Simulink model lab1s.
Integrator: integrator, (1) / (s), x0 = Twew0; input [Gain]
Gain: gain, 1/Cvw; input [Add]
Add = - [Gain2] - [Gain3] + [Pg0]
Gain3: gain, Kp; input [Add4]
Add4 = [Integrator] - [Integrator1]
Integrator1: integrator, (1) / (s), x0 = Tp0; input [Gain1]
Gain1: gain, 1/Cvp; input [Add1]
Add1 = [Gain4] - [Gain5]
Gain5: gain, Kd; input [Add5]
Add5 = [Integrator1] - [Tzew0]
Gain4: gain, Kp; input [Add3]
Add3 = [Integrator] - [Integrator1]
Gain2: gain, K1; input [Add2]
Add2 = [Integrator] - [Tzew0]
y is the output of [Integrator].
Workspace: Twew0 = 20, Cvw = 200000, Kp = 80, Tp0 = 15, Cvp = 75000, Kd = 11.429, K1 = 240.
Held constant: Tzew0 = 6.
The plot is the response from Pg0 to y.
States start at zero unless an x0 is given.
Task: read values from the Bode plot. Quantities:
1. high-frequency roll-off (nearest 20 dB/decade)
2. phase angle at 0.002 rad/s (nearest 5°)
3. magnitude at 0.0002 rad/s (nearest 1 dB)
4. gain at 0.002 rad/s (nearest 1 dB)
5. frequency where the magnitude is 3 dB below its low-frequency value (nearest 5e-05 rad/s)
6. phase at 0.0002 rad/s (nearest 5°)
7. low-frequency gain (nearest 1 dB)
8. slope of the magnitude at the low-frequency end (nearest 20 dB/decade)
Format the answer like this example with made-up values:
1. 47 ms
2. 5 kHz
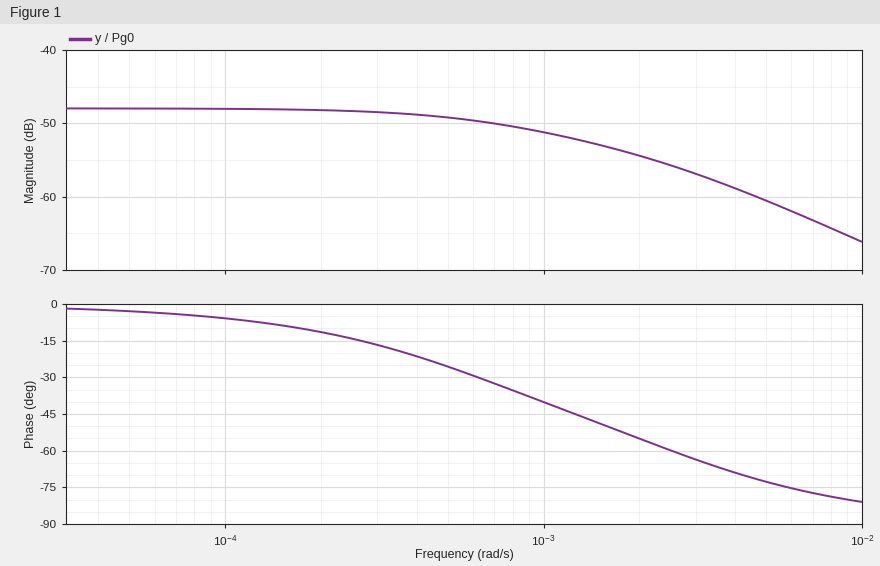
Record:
1. -20 dB/decade
2. -55°
3. -48 dB
4. -54 dB
5. 0.00095 rad/s
6. -10°
7. -48 dB
8. 0 dB/decade
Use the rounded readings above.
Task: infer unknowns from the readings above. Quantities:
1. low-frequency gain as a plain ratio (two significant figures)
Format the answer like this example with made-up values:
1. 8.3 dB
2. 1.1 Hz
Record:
1. 0.0040
